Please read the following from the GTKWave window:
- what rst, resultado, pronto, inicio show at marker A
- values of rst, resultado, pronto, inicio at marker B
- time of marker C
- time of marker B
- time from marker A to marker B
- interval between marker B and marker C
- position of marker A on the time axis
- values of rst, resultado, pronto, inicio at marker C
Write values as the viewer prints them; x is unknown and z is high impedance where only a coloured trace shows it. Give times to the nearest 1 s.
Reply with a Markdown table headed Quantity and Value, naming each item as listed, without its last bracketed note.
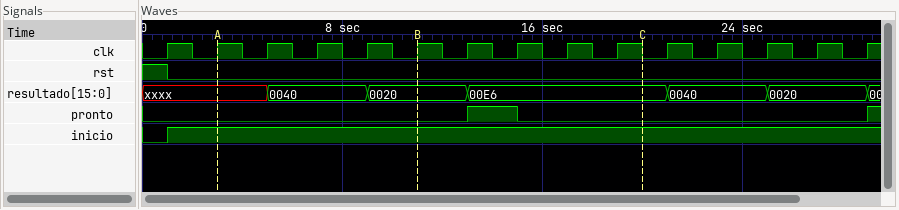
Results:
| Quantity | Value |
|---|---|
| what rst, resultado, pronto, inicio show at marker A | rst=0, resultado=xxxx, pronto=0, inicio=1 |
| values of rst, resultado, pronto, inicio at marker B | rst=0, resultado=0020, pronto=0, inicio=1 |
| time of marker C | 20 s |
| time of marker B | 11 s |
| time from marker A to marker B | 8 s |
| interval between marker B and marker C | 9 s |
| position of marker A on the time axis | 3 s |
| values of rst, resultado, pronto, inicio at marker C | rst=0, resultado=00E6, pronto=0, inicio=1 |
